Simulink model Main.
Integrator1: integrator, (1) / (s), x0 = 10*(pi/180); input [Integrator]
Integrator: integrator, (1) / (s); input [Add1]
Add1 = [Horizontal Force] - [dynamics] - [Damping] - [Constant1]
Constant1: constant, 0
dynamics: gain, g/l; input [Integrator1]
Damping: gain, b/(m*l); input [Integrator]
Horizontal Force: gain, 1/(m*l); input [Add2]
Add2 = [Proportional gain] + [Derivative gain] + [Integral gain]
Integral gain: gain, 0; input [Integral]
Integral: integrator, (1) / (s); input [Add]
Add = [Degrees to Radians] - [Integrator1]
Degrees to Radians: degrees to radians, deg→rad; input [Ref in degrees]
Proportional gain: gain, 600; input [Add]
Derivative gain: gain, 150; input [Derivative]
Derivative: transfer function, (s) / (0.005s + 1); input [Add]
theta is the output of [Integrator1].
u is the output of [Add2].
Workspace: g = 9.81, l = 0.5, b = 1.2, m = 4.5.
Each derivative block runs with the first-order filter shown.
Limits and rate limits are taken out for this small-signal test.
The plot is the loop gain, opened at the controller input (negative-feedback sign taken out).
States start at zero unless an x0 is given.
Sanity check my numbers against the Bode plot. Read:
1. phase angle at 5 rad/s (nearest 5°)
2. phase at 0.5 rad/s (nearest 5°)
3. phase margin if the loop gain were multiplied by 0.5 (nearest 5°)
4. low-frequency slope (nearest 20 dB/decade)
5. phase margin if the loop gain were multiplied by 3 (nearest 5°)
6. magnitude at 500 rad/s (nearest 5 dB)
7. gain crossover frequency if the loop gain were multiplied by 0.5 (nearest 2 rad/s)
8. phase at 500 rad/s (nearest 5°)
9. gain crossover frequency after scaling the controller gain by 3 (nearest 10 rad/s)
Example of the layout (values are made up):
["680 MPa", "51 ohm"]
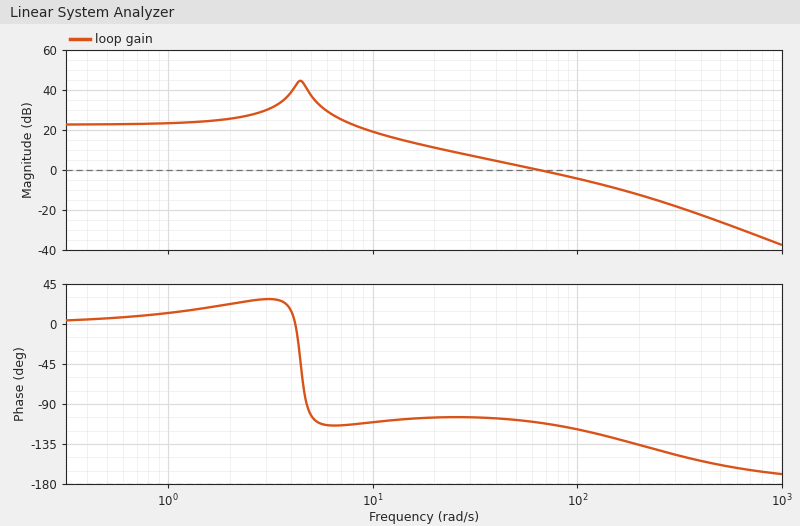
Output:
["-105°", "5°", "75°", "0 dB/decade", "50°", "-25 dB", "34 rad/s", "-160°", "160 rad/s"]
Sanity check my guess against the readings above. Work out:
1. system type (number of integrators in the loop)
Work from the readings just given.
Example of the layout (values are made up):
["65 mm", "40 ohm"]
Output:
["0"]
